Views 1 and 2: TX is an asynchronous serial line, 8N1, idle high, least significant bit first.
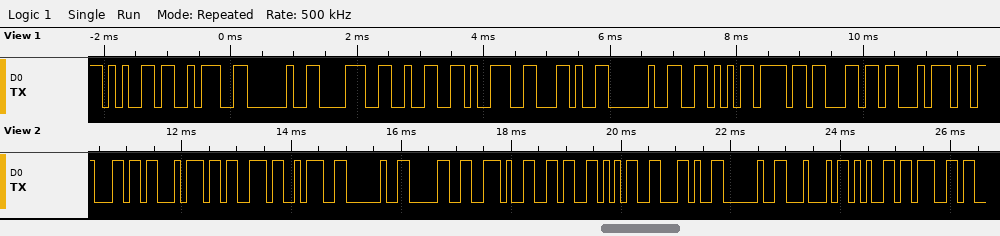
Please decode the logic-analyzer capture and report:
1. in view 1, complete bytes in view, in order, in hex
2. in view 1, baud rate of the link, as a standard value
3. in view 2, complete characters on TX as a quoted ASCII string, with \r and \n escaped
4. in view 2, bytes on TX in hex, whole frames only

65 3A 20 38 32 39 2C 20 56 6F 6C 74
9600 baud
"lts: 0.65, Deg"
6C 74 73 3A 20 30 2E 36 35 2C 20 44 65 67
